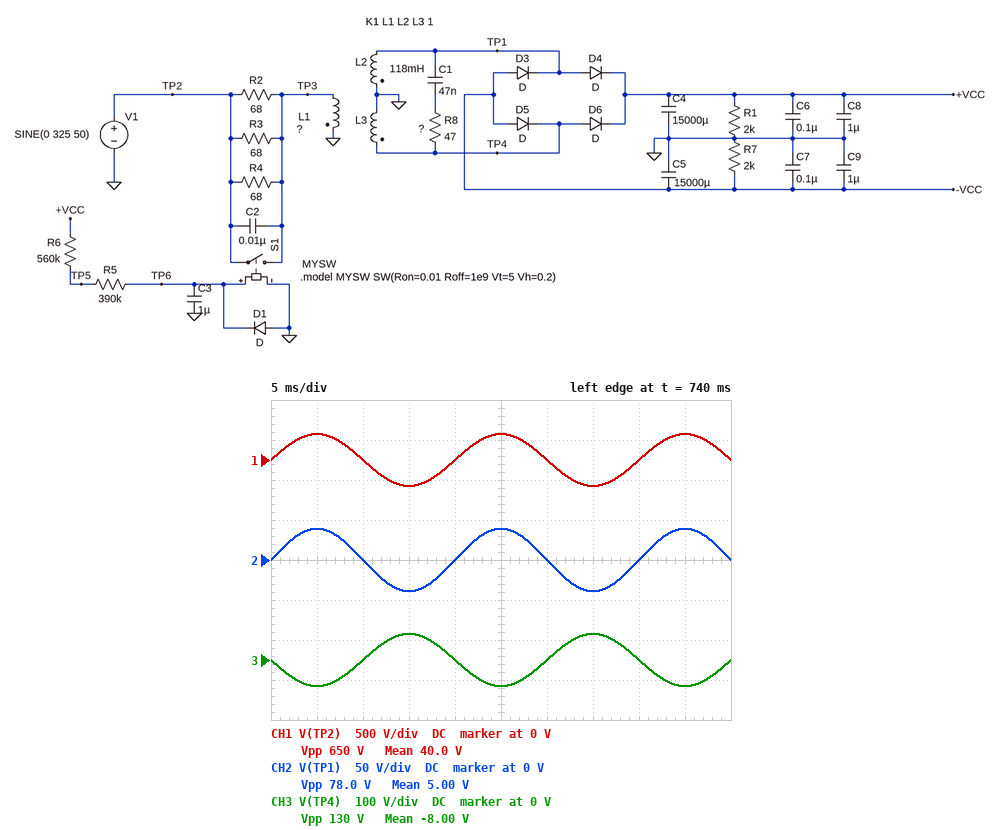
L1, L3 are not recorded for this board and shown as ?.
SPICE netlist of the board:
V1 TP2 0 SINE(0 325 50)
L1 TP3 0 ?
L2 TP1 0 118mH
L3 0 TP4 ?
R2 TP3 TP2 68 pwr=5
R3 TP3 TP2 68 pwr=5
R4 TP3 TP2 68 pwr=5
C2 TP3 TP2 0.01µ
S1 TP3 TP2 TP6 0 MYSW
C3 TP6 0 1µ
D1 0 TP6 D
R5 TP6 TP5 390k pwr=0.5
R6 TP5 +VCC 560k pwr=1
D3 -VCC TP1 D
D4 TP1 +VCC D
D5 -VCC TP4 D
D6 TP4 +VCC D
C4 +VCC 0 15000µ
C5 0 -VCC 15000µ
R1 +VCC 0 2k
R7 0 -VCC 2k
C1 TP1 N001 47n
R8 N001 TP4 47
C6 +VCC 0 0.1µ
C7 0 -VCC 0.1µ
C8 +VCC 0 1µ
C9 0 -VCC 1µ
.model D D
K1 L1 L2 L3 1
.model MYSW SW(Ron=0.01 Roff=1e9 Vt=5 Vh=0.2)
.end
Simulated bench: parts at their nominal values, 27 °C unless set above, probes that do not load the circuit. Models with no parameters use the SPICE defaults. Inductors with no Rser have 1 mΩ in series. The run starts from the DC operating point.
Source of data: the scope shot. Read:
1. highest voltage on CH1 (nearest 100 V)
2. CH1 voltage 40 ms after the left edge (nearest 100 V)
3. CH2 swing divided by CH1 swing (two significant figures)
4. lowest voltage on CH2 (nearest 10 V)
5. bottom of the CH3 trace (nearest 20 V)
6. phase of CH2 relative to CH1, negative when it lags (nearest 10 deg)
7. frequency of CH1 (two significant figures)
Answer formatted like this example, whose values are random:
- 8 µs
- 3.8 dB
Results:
- 300 V
- 0 V
- 0.12
- -40 V
- -60 V
- 0 deg
- 50 Hz
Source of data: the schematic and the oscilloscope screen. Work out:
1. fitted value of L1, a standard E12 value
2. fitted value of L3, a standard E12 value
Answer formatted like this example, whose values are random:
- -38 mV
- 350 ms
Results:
- 8.2 H
- 330 mH
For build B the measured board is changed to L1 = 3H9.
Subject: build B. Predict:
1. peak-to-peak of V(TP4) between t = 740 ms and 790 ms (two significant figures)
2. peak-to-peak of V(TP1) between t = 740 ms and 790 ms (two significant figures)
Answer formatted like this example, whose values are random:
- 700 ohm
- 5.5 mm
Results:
- 190 V
- 110 V
